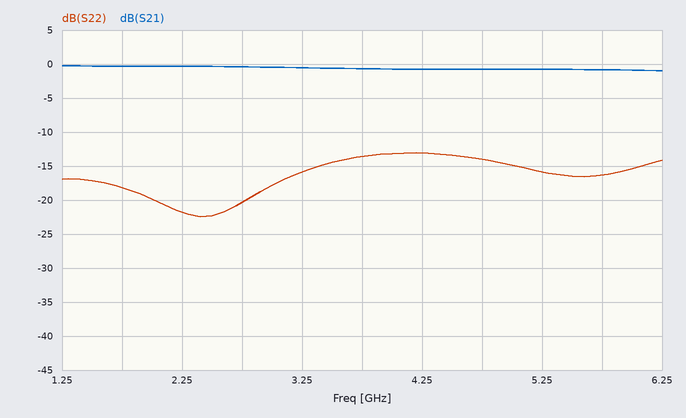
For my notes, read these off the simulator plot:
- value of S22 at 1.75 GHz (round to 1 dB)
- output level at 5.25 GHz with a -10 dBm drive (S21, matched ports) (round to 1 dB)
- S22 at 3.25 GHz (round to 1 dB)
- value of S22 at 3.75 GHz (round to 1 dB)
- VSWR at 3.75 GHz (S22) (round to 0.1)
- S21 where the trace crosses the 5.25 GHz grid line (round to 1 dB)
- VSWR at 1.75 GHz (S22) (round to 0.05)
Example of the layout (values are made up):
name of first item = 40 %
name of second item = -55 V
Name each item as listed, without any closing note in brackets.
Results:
value of S22 at 1.75 GHz = -18 dB
output level at 5.25 GHz with a -10 dBm drive (S21, matched ports) = -11 dBm
S22 at 3.25 GHz = -16 dB
value of S22 at 3.75 GHz = -14 dB
VSWR at 3.75 GHz (S22) = 1.5
S21 where the trace crosses the 5.25 GHz grid line = -1 dB
VSWR at 1.75 GHz (S22) = 1.30
